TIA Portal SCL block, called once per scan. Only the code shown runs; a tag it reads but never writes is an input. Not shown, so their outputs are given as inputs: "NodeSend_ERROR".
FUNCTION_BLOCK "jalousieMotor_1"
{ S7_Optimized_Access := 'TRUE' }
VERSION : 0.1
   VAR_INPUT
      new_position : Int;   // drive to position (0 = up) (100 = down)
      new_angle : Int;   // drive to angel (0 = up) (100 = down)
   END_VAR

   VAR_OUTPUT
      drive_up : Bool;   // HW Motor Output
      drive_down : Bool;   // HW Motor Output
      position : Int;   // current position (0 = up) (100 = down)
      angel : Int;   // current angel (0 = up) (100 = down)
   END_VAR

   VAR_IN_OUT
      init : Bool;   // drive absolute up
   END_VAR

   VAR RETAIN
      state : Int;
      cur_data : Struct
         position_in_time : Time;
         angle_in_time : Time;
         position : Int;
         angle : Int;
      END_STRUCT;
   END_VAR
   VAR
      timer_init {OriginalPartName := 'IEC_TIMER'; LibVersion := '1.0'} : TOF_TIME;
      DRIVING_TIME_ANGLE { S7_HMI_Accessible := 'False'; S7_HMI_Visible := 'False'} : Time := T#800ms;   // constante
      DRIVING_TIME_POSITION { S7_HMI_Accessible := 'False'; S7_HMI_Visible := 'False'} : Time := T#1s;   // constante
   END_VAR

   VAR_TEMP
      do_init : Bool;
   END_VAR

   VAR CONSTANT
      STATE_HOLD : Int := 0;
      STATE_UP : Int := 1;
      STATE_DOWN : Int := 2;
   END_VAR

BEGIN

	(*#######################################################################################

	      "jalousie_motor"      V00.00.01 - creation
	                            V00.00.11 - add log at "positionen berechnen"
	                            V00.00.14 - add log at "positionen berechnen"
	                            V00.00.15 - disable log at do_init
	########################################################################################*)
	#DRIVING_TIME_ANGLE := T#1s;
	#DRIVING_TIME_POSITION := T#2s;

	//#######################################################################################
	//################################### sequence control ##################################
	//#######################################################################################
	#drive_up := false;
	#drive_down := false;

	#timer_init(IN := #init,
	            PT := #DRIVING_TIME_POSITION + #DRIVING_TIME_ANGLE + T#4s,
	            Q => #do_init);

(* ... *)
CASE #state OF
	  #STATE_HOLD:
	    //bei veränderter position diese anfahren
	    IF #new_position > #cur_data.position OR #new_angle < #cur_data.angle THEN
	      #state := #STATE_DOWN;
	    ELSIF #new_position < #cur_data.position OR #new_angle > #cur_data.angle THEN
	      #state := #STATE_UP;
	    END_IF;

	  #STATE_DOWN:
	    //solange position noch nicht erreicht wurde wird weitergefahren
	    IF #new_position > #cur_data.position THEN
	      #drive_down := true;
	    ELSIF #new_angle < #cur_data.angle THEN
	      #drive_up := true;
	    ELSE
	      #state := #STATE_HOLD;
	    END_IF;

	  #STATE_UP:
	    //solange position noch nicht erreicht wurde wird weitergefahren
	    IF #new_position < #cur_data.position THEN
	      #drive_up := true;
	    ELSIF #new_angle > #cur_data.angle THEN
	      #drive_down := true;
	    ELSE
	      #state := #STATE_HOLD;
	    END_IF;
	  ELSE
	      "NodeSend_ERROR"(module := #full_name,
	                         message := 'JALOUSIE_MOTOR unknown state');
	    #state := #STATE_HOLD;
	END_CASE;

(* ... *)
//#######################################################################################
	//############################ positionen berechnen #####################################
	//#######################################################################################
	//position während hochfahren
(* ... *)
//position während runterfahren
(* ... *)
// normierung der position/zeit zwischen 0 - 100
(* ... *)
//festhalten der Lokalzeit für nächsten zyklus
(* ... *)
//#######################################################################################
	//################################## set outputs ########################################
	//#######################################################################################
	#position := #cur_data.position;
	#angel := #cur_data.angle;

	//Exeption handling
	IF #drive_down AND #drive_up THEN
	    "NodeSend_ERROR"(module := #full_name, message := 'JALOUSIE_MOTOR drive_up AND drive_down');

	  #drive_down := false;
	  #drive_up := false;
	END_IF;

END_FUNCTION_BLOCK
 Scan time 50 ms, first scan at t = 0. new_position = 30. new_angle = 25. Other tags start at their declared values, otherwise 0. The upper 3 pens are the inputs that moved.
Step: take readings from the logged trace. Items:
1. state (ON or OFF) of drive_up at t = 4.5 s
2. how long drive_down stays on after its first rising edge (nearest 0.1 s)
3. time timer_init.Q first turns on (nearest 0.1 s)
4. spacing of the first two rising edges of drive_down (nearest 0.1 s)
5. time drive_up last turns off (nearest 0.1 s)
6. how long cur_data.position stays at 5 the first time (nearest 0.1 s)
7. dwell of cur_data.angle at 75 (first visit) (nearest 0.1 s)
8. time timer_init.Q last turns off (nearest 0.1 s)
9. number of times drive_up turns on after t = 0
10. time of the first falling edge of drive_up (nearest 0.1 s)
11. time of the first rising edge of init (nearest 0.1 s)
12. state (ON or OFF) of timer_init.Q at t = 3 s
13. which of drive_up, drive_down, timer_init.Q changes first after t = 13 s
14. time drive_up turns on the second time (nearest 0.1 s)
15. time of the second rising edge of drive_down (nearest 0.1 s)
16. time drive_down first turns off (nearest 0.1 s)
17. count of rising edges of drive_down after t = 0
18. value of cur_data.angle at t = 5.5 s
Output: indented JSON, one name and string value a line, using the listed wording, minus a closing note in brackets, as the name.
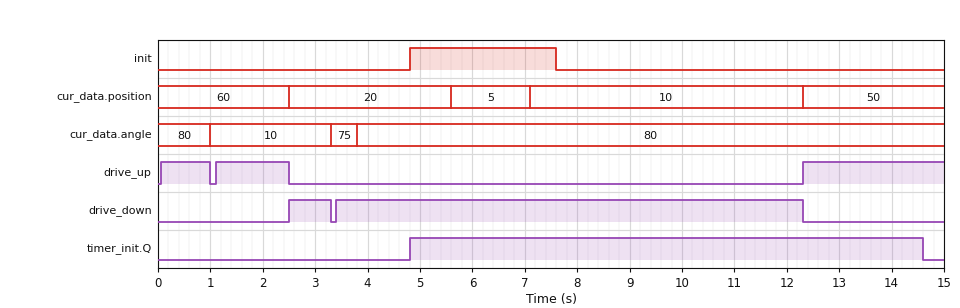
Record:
{
  "state (ON or OFF) of drive_up at t = 4.5 s": "OFF",
  "how long drive_down stays on after its first rising edge": "0.8 s",
  "time timer_init.Q first turns on": "4.8 s",
  "spacing of the first two rising edges of drive_down": "0.9 s",
  "time drive_up last turns off": "2.5 s",
  "how long cur_data.position stays at 5 the first time": "1.5 s",
  "dwell of cur_data.angle at 75 (first visit)": "0.5 s",
  "time timer_init.Q last turns off": "14.6 s",
  "number of times drive_up turns on after t = 0": "3",
  "time of the first falling edge of drive_up": "1.0 s",
  "time of the first rising edge of init": "4.8 s",
  "state (ON or OFF) of timer_init.Q at t = 3 s": "OFF",
  "which of drive_up, drive_down, timer_init.Q changes first after t = 13 s": "timer_init.Q",
  "time drive_up turns on the second time": "1.1 s",
  "time of the second rising edge of drive_down": "3.4 s",
  "time drive_down first turns off": "3.3 s",
  "count of rising edges of drive_down after t = 0": "2",
  "value of cur_data.angle at t = 5.5 s": "80"
}
